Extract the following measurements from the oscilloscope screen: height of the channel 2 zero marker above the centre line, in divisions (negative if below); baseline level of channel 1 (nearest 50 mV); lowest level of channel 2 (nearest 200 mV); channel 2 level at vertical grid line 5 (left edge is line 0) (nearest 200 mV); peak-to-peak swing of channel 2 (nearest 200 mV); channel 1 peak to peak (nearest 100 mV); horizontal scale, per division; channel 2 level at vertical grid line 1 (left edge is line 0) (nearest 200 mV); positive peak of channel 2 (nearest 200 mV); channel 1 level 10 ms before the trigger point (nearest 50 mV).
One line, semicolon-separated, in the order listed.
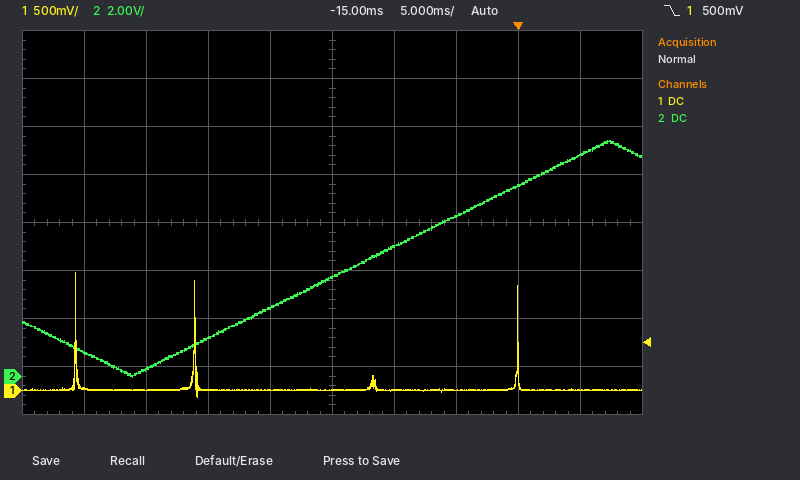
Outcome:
-3.2 div; 0 mV; 0.0 V; 4.2 V; 9.8 V; 1.30 V; 5 ms; 1.0 V; 9.8 V; 0 mV
